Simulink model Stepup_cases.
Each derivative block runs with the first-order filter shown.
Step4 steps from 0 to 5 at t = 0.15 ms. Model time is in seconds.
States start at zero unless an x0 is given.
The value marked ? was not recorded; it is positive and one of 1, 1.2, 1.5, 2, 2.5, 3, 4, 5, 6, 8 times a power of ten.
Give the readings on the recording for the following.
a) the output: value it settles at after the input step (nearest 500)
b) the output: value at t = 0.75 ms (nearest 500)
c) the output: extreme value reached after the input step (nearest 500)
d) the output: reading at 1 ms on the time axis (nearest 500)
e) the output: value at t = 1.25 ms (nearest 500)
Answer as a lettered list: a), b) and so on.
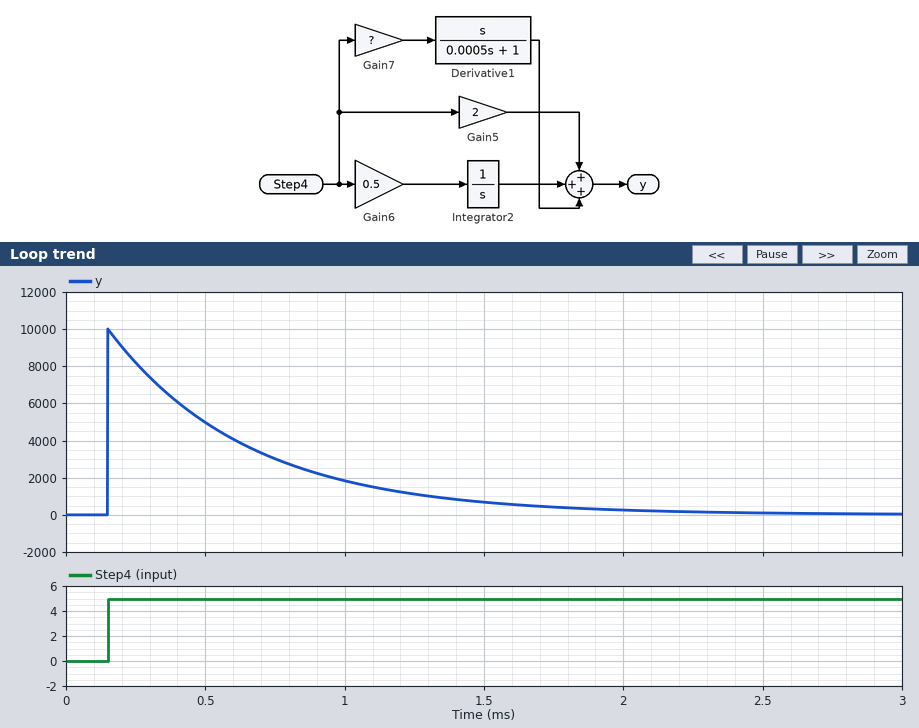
a) 0
b) 3000
c) 10000
d) 2000
e) 1000
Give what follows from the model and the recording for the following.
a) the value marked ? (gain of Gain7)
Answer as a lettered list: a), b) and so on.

a) 1
